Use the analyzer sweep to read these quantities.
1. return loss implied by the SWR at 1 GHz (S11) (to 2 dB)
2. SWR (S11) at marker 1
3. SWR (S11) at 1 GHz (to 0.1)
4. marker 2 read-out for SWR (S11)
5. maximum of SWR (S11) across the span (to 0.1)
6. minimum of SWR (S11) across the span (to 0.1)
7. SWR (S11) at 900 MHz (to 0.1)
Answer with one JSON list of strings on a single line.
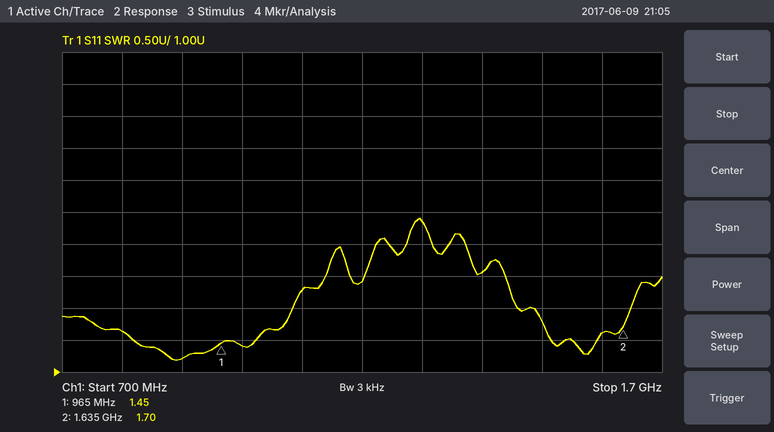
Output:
["16 dB", "1.45", "1.4", "1.70", "3.4", "1.2", "1.2"]
